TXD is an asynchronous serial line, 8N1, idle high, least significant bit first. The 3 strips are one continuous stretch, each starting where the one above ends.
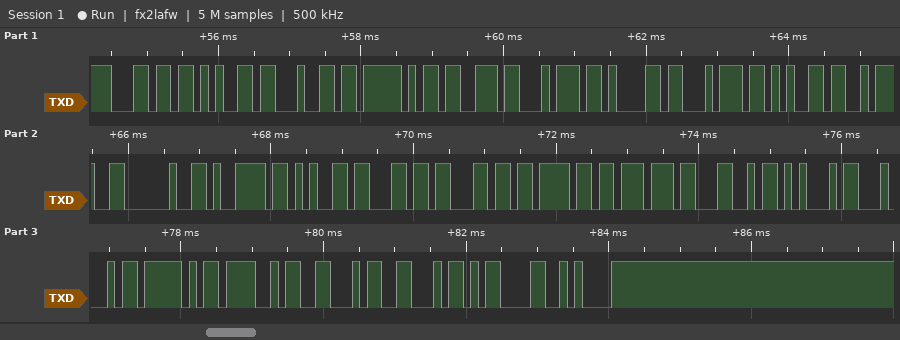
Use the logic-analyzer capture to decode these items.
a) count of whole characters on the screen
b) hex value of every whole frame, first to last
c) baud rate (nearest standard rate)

26
6C 65 64 5F 73 74 61 74 65 3A 20 79 65 6C 6C 6F 77 4C 45 44 5F 4F 46 46 0D 0A
9600 baud
